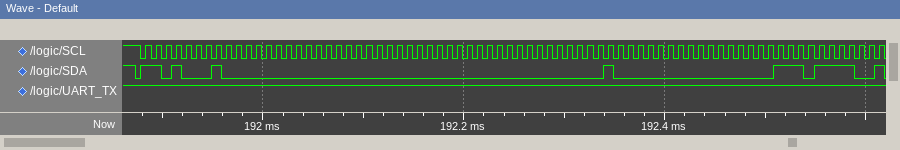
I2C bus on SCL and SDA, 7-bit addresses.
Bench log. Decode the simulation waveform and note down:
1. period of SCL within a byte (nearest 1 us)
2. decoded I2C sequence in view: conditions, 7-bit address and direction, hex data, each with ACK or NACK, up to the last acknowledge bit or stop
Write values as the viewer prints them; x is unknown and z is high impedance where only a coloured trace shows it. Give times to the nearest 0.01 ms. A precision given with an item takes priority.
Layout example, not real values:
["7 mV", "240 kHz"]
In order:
["10 us", "start, address 68 read ACK, 00 ACK, 00 ACK, 00 ACK, 00 ACK, 40 ACK, 00 ACK, EF ACK"]
